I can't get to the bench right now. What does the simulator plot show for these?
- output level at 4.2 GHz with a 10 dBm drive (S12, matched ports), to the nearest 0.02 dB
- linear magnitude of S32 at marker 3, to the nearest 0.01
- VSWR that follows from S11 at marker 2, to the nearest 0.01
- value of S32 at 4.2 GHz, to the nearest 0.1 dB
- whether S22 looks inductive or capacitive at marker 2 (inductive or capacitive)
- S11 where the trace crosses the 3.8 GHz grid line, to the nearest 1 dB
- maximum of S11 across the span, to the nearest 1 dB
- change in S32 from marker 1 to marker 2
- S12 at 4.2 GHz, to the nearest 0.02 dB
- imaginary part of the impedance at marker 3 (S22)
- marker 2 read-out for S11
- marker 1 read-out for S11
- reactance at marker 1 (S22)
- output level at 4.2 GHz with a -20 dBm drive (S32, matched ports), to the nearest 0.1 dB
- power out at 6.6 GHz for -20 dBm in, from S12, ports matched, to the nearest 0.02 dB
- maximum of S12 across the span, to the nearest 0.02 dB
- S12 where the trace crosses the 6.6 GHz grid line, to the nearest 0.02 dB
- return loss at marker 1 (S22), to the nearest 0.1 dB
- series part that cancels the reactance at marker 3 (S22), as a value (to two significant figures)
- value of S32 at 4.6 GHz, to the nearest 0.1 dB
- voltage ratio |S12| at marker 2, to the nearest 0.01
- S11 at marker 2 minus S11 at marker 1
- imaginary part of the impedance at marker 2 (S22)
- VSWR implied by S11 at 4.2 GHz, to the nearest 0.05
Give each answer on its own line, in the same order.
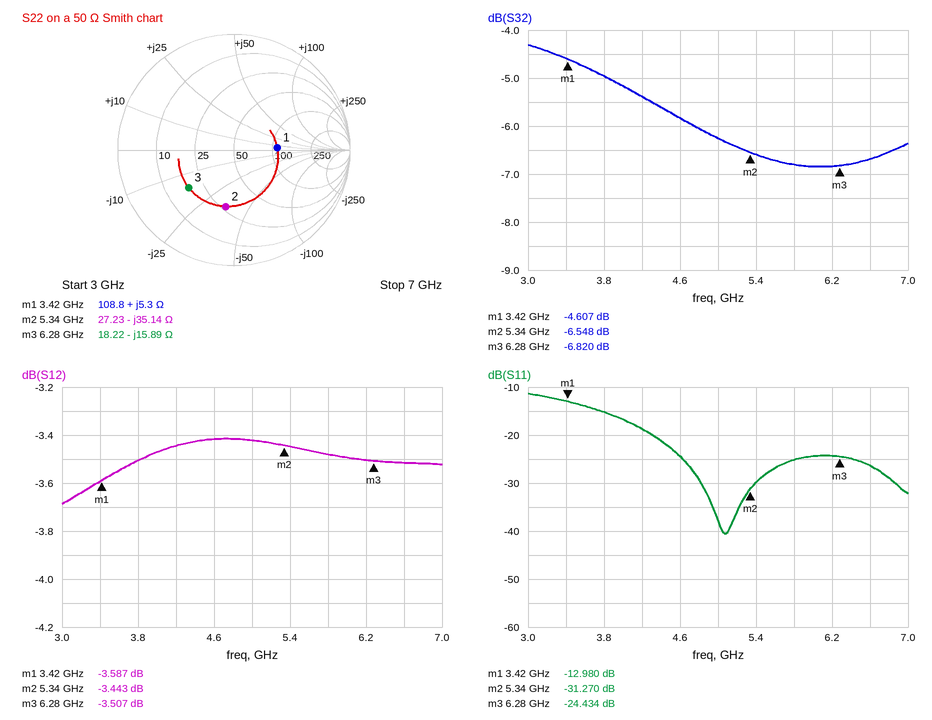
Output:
6.56 dBm
0.46
1.06
-5.4 dB
capacitive
-15 dB
-11 dB
-1.941 dB
-3.44 dB
-15.89 Ω
-31.270 dB
-12.980 dB
+5.3 Ω
-25.4 dBm
-23.52 dBm
-3.42 dB
-3.52 dB
8.6 dB
400 pH
-5.8 dB
0.67
-18.290 dB
-35.14 Ω
1.25
